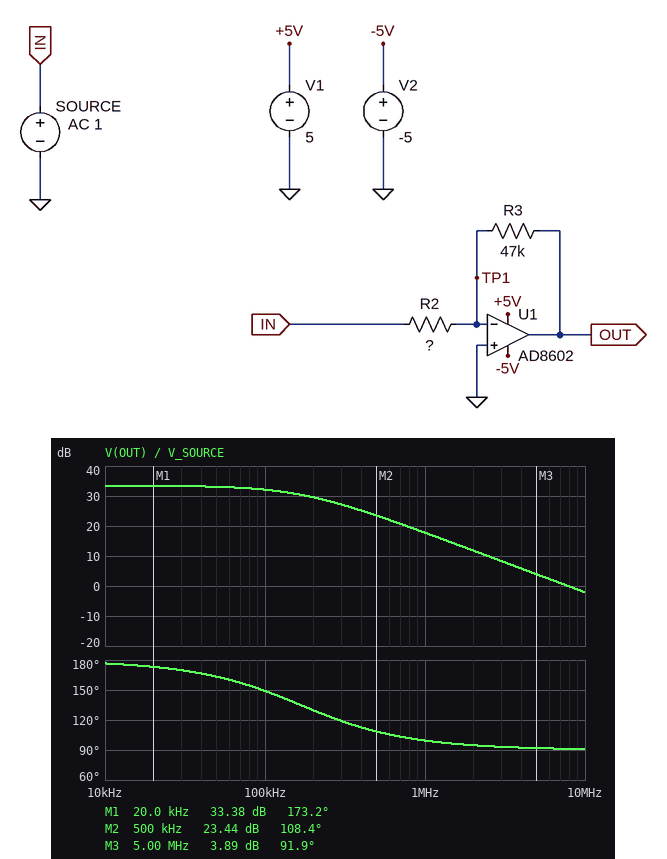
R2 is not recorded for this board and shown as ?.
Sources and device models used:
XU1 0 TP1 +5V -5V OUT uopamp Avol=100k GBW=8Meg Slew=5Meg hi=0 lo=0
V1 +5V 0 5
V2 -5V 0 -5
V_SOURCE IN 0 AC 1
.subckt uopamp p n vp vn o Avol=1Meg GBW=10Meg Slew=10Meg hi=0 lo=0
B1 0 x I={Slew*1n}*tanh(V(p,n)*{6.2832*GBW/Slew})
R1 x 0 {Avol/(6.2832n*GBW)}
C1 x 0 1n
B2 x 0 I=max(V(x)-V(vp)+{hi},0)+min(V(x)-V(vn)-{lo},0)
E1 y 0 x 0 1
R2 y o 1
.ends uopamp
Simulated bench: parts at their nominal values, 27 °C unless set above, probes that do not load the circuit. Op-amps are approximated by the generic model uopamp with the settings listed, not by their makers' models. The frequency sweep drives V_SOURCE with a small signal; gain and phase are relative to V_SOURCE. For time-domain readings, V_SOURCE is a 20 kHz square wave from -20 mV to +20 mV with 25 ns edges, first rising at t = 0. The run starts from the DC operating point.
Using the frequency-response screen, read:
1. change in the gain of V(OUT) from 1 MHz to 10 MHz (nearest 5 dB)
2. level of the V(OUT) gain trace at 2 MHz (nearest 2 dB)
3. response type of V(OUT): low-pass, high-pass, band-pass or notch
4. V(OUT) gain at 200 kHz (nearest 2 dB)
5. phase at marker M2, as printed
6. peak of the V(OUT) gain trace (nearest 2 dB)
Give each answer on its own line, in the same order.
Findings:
-20 dB
12 dB
low-pass
30 dB
108.4 deg
34 dB
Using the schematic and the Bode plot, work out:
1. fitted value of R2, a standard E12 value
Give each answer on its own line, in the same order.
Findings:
1 kΩ
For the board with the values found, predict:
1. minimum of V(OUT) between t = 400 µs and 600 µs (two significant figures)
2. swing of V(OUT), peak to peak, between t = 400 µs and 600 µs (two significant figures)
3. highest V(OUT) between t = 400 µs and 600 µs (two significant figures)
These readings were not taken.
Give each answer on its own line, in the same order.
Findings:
-940 mV
1.9 V
940 mV
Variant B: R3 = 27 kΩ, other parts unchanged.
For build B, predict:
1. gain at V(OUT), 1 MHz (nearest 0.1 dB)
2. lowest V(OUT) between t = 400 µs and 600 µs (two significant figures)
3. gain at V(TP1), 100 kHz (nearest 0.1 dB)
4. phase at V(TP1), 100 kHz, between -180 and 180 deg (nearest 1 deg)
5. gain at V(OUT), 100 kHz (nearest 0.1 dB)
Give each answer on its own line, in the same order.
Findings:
17.4 dB
-540 mV
-9.9 dB
71 deg
28.1 dB
